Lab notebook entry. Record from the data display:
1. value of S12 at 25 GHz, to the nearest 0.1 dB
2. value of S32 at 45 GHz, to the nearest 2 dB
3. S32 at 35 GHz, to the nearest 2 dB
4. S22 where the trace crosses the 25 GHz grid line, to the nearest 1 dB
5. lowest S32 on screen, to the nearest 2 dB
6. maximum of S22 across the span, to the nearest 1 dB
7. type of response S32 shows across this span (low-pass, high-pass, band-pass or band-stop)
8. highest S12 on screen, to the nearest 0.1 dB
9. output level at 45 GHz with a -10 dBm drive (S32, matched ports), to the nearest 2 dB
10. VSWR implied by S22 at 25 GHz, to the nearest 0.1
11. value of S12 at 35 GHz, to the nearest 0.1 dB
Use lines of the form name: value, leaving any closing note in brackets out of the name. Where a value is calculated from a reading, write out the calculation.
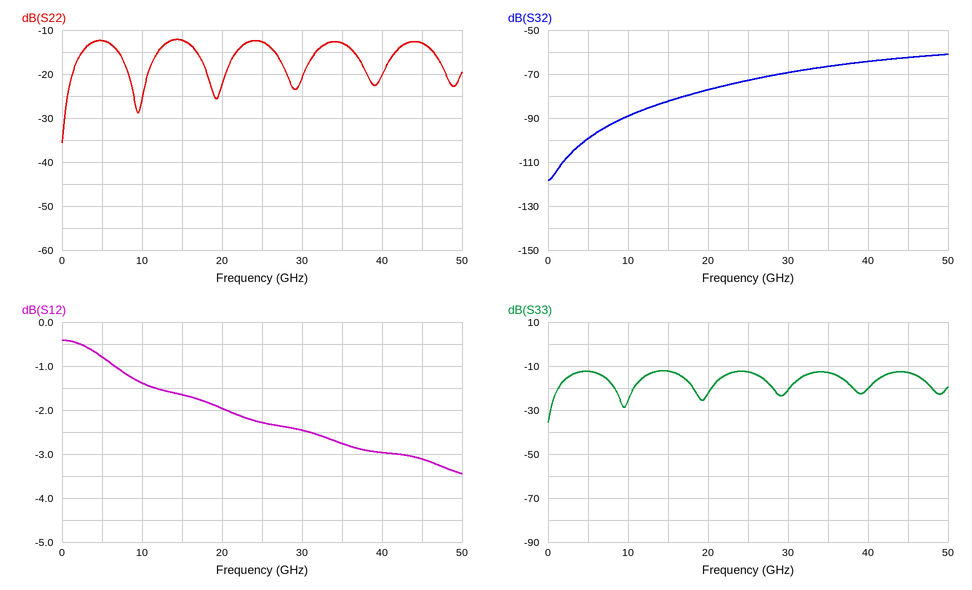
value of S12 at 25 GHz, to the nearest 0.1 dB: -2.3 dB
value of S32 at 45 GHz, to the nearest 2 dB: -62 dB
S32 at 35 GHz, to the nearest 2 dB: -66 dB
S22 where the trace crosses the 25 GHz grid line, to the nearest 1 dB: -13 dB
lowest S32 on screen, to the nearest 2 dB: -118 dB
maximum of S22 across the span, to the nearest 1 dB: -12 dB
type of response S32 shows across this span: high-pass
highest S12 on screen, to the nearest 0.1 dB: -0.4 dB
output level at 45 GHz with a -10 dBm drive (S32, matched ports), to the nearest 2 dB: -10 dBm + (-62 dB) = -72 dBm
VSWR implied by S22 at 25 GHz, to the nearest 0.1: |Γ| = 10^(-13/20) = 0.2239; VSWR = (1 + 0.2239)/(1 − 0.2239) ≈ 1.6
value of S12 at 35 GHz, to the nearest 0.1 dB: -2.8 dB
